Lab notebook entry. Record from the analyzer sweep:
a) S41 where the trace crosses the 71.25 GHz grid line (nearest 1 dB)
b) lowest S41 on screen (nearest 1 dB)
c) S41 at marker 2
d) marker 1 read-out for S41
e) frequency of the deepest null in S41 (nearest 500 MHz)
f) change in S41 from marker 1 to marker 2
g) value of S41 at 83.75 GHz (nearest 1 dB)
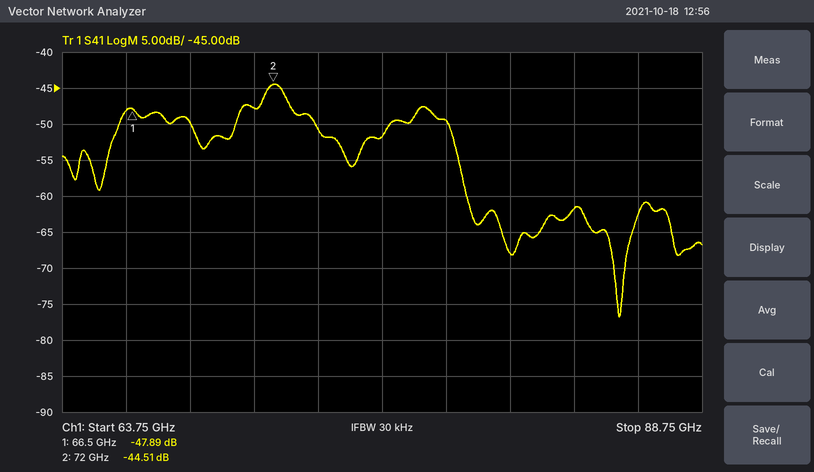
-48 dB
-77 dB
-44.51 dB
-47.89 dB
85.5 GHz
3.38 dB
-62 dB
